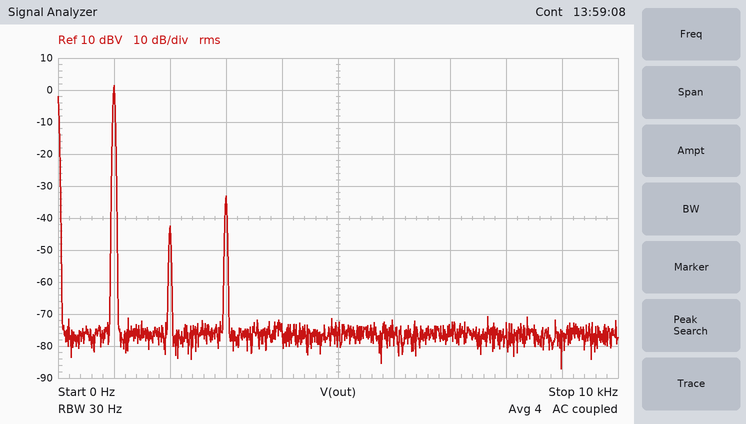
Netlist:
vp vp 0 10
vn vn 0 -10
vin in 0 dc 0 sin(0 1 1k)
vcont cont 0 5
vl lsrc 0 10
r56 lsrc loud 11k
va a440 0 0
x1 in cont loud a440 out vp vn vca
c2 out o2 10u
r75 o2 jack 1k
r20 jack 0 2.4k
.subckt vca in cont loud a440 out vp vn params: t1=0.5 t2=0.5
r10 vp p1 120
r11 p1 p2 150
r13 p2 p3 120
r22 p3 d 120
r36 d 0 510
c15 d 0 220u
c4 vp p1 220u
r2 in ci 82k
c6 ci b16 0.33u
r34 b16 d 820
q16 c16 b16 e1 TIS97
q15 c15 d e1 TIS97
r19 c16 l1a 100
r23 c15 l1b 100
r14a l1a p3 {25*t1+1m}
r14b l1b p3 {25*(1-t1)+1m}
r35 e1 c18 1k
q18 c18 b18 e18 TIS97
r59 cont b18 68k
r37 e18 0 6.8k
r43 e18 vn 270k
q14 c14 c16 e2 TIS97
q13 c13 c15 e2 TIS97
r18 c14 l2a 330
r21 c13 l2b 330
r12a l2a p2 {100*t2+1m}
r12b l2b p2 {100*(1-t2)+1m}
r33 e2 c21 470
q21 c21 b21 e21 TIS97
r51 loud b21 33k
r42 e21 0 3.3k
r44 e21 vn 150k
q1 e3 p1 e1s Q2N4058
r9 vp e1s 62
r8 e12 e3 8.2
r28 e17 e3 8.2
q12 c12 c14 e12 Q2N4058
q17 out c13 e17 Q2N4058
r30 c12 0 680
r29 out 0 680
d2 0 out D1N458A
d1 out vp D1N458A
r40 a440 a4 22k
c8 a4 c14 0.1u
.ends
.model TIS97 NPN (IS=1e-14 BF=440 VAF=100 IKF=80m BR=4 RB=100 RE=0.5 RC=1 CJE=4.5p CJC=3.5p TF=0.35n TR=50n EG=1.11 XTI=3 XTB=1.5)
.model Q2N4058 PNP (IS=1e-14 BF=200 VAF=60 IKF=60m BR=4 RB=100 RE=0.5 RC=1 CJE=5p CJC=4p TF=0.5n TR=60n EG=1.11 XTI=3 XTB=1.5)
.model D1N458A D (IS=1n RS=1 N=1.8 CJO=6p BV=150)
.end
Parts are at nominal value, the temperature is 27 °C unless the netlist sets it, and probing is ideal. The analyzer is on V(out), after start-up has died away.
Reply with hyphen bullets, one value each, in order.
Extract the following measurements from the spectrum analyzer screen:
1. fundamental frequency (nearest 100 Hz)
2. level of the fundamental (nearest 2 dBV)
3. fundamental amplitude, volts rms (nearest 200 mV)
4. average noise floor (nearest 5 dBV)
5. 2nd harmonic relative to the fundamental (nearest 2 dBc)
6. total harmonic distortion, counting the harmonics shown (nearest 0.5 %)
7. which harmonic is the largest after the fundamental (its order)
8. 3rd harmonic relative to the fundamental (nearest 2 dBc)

- 1.0 kHz
- 2 dBV
- 1.2 V
- -75 dBV
- -44 dBc
- 2.0 %
- 3
- -34 dBc
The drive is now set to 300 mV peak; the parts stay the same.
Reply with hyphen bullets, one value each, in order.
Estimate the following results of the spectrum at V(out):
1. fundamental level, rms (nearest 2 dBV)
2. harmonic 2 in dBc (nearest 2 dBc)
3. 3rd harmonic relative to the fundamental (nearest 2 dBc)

- -8 dBV
- -54 dBc
- -56 dBc
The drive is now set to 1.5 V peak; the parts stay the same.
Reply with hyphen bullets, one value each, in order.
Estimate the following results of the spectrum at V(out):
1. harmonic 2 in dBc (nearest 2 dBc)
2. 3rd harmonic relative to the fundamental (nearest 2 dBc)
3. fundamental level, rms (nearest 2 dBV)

- -40 dBc
- -26 dBc
- 4 dBV
